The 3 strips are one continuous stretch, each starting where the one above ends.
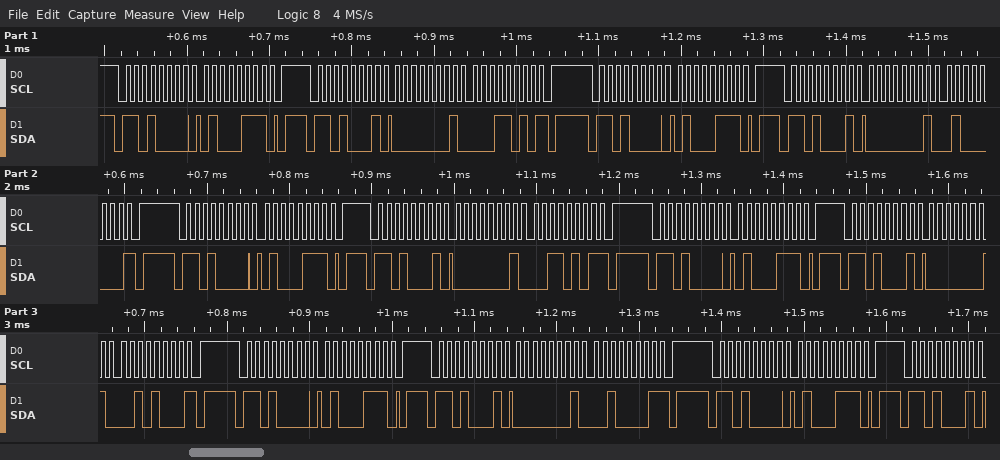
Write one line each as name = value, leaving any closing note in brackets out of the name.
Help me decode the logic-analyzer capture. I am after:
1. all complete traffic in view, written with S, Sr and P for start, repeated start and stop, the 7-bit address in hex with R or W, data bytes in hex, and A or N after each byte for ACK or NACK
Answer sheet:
all complete traffic in view, written with S, Sr and P for start, repeated start and stop, the 7-bit address in hex with R or W, data bytes in hex, and A or N after each byte for ACK or NACK = S 68W A 47 A P S 68R A 01 A 1A N P S 68W A 47 A P S 68R A 01 A 40 N P S 68W A 47 A P S 68R A 01 A 35 N P S 68W A 47 A P S 68R A 01 A 28 N P S 68W A 47 A P S 68R A 01 A 21 N P S 68W A 47 A P S 68R A
